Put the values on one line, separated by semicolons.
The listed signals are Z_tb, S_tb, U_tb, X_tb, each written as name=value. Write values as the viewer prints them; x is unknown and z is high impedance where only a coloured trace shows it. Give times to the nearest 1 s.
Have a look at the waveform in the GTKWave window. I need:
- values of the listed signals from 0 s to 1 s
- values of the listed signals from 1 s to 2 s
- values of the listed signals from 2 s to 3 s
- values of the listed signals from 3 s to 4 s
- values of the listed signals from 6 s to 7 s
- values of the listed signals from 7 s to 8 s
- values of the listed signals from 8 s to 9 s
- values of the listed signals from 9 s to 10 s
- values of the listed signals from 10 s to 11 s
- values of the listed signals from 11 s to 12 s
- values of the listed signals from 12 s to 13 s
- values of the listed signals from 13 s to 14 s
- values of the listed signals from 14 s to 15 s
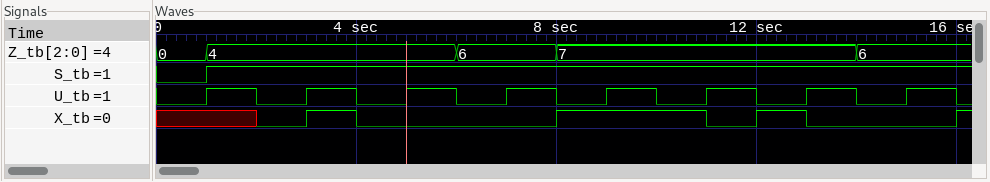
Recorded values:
Z_tb=0, S_tb=0, U_tb=0, X_tb=x; Z_tb=4, S_tb=1, U_tb=1, X_tb=x; Z_tb=4, S_tb=1, U_tb=0, X_tb=0; Z_tb=4, S_tb=1, U_tb=1, X_tb=1; Z_tb=6, S_tb=1, U_tb=0, X_tb=0; Z_tb=6, S_tb=1, U_tb=1, X_tb=0; Z_tb=7, S_tb=1, U_tb=0, X_tb=1; Z_tb=7, S_tb=1, U_tb=1, X_tb=1; Z_tb=7, S_tb=1, U_tb=0, X_tb=1; Z_tb=7, S_tb=1, U_tb=1, X_tb=0; Z_tb=7, S_tb=1, U_tb=0, X_tb=1; Z_tb=7, S_tb=1, U_tb=1, X_tb=0; Z_tb=6, S_tb=1, U_tb=0, X_tb=0
